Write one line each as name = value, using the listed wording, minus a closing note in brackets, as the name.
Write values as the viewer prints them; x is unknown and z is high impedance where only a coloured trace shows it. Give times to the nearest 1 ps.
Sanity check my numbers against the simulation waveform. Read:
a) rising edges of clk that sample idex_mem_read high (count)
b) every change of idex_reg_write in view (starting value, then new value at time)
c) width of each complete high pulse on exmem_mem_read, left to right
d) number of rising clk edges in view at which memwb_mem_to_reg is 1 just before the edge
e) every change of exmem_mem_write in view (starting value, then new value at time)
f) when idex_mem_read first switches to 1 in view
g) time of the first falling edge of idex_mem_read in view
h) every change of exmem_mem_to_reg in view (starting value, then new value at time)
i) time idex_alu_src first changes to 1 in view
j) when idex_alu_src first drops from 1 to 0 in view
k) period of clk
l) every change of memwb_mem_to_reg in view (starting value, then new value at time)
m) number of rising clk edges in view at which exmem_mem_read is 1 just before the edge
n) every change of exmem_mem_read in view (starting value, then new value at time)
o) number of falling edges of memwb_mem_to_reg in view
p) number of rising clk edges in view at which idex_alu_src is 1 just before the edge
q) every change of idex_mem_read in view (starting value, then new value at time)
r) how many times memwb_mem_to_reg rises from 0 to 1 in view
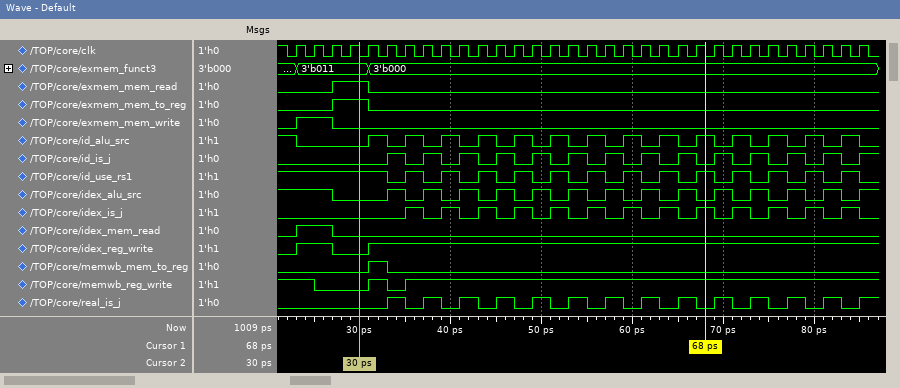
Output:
rising edges of clk that sample idex_mem_read high = 2
every change of idex_reg_write in view = 0, 1 at 23 ps, 0 at 27 ps, 1 at 31 ps
width of each complete high pulse on exmem_mem_read, left to right = 4 ps
number of rising clk edges in view at which memwb_mem_to_reg is 1 just before the edge = 1
every change of exmem_mem_write in view = 0, 1 at 23 ps, 0 at 27 ps
when idex_mem_read first switches to 1 in view = 23 ps
time of the first falling edge of idex_mem_read in view = 27 ps
every change of exmem_mem_to_reg in view = 0, 1 at 27 ps, 0 at 31 ps
time idex_alu_src first changes to 1 in view = 33 ps
when idex_alu_src first drops from 1 to 0 in view = 27 ps
period of clk = 2 ps
every change of memwb_mem_to_reg in view = 0, 1 at 31 ps, 0 at 33 ps
number of rising clk edges in view at which exmem_mem_read is 1 just before the edge = 2
every change of exmem_mem_read in view = 0, 1 at 27 ps, 0 at 31 ps
number of falling edges of memwb_mem_to_reg in view = 1
number of rising clk edges in view at which idex_alu_src is 1 just before the edge = 16
every change of idex_mem_read in view = 0, 1 at 23 ps, 0 at 27 ps
how many times memwb_mem_to_reg rises from 0 to 1 in view = 1
